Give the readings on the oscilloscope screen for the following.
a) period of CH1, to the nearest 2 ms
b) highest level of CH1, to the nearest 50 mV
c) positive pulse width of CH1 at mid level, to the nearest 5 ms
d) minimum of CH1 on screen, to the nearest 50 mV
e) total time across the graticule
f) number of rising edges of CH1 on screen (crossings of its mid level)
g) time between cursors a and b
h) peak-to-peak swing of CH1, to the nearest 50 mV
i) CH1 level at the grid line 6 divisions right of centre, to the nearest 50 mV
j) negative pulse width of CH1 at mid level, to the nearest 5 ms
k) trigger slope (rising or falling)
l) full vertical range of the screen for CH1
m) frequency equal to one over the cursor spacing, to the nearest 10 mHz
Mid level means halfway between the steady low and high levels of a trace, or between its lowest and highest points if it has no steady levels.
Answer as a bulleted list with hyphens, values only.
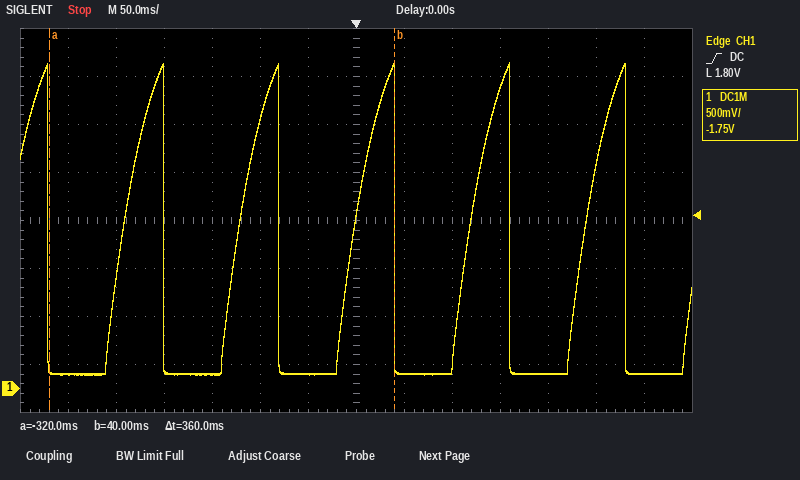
- 120 ms
- 3.40 V
- 40 ms
- 150 mV
- 700 ms
- 5
- 360 ms
- 3.25 V
- 150 mV
- 80 ms
- rising
- 4 V
- 2.78 Hz
